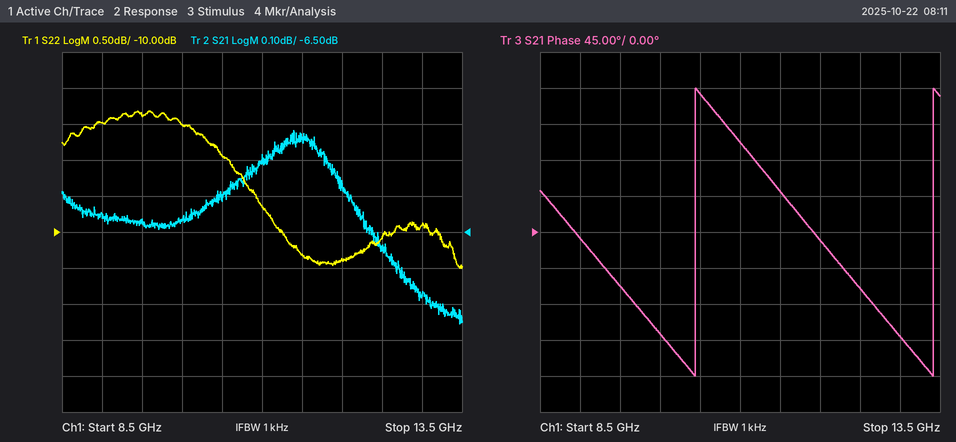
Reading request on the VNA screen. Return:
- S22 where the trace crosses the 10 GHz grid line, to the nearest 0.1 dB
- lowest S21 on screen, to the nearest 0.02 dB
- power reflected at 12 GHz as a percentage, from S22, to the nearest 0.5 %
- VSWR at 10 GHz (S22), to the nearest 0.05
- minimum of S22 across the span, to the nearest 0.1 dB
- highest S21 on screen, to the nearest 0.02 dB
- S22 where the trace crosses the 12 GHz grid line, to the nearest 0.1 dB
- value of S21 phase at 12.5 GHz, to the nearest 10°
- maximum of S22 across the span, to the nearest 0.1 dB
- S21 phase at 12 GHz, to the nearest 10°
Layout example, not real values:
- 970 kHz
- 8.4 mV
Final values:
- -8.5 dB
- -6.76 dB
- 9.0 %
- 2.20
- -10.5 dB
- -6.22 dB
- -10.4 dB
- -70°
- -8.3 dB
- -10°
